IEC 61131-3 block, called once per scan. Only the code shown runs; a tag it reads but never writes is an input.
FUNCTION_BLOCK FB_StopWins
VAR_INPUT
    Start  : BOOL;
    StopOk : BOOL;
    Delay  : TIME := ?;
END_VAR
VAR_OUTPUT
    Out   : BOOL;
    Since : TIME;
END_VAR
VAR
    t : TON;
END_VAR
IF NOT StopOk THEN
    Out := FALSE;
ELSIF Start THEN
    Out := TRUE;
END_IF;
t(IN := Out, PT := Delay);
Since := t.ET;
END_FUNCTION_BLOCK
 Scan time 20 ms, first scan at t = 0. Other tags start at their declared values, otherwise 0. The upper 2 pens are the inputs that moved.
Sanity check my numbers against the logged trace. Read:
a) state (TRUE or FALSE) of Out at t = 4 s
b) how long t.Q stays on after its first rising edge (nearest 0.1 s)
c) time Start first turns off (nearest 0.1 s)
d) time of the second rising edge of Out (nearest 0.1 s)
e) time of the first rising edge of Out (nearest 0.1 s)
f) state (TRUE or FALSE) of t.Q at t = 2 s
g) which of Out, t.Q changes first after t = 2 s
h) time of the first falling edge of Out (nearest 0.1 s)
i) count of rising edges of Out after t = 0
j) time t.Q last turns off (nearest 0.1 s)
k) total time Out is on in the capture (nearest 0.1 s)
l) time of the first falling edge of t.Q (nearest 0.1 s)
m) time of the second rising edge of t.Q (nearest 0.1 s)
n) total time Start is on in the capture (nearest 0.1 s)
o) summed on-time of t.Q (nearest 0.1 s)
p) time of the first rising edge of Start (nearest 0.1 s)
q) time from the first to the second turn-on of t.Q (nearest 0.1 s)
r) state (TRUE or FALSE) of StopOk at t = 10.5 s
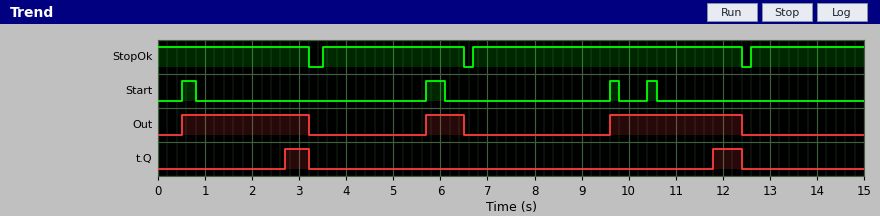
FALSE
0.5 s
0.8 s
5.7 s
0.5 s
FALSE
t.Q
3.2 s
3
12.4 s
6.3 s
3.2 s
11.8 s
1.1 s
1.1 s
0.5 s
9.1 s
TRUE
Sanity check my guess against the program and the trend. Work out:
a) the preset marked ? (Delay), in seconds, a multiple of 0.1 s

2.2 s
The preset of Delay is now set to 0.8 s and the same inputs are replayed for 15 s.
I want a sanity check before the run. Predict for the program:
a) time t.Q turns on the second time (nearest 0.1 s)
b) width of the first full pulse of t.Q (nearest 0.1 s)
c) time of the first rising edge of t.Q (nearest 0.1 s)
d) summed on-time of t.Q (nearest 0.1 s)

10.4 s
1.9 s
1.3 s
3.9 s
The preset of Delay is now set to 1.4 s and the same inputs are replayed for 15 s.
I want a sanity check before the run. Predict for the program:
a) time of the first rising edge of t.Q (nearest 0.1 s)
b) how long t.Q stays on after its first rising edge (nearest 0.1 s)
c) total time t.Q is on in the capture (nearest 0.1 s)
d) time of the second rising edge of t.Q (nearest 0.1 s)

1.9 s
1.3 s
2.7 s
11.0 s
